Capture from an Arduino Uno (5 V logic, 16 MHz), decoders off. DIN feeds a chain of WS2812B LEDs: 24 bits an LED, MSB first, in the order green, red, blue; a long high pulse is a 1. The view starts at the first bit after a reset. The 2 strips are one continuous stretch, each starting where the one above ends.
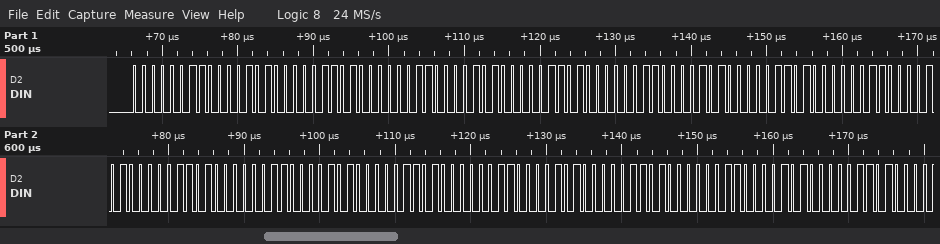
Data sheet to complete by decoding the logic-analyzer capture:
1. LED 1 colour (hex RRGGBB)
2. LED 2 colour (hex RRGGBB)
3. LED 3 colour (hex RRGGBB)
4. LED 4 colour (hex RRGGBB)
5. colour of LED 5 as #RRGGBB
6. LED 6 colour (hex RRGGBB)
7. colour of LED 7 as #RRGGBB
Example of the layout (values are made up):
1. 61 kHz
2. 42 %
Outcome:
1. #0A030D
2. #0A030D
3. #0A030D
4. #0A030D
5. #0A030D
6. #0A030D
7. #0A030D
